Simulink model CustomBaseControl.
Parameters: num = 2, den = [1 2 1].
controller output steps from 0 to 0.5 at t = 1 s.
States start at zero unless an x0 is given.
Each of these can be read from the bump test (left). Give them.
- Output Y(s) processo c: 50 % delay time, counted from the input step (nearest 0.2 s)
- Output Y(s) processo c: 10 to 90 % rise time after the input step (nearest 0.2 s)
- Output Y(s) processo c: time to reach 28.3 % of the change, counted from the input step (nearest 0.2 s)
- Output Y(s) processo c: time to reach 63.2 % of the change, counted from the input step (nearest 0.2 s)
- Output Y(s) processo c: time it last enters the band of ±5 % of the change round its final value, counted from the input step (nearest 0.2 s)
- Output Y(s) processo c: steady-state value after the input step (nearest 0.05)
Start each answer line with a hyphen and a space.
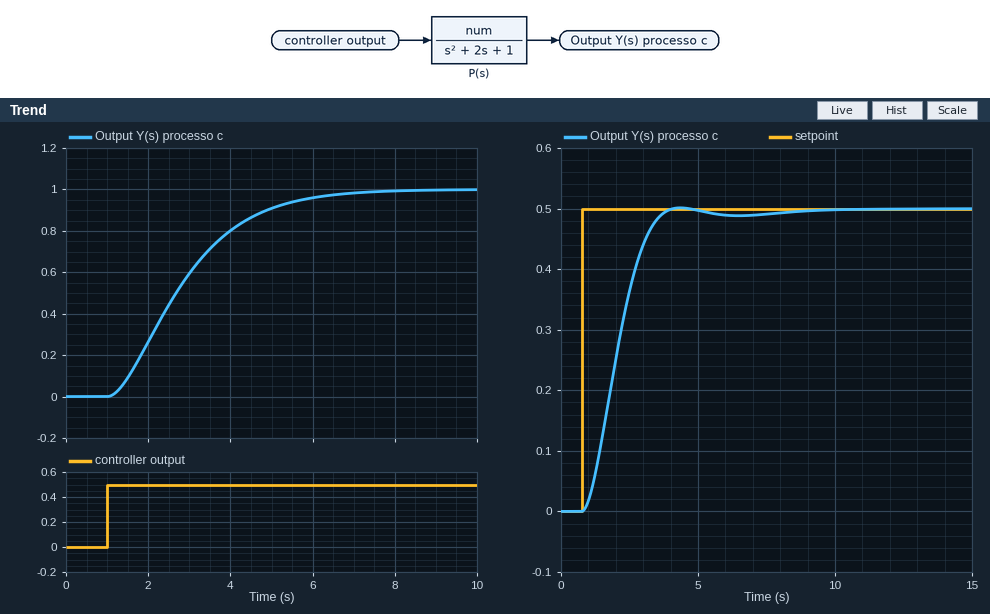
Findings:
- 1.6 s
- 3.4 s
- 1.0 s
- 2.2 s
- 4.8 s
- 1.00
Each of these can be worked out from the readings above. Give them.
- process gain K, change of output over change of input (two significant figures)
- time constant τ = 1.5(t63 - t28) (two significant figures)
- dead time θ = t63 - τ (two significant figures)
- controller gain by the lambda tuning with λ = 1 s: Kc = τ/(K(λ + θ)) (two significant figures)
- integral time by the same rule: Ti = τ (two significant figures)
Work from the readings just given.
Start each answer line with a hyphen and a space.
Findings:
- 2.0
- 1.8 s
- 0.40 s
- 0.64
- 1.8 s
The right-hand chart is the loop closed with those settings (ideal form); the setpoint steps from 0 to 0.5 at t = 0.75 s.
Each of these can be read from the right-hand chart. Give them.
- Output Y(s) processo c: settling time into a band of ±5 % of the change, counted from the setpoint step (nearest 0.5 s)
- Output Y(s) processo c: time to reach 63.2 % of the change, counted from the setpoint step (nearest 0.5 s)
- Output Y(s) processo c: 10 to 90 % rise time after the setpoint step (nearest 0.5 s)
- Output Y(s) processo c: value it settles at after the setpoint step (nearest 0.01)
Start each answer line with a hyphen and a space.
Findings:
- 2.5 s
- 1.5 s
- 2.0 s
- 0.50
